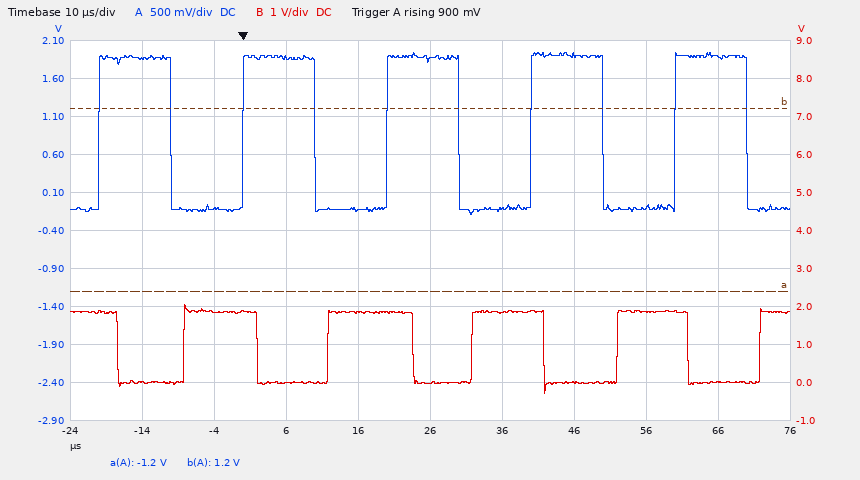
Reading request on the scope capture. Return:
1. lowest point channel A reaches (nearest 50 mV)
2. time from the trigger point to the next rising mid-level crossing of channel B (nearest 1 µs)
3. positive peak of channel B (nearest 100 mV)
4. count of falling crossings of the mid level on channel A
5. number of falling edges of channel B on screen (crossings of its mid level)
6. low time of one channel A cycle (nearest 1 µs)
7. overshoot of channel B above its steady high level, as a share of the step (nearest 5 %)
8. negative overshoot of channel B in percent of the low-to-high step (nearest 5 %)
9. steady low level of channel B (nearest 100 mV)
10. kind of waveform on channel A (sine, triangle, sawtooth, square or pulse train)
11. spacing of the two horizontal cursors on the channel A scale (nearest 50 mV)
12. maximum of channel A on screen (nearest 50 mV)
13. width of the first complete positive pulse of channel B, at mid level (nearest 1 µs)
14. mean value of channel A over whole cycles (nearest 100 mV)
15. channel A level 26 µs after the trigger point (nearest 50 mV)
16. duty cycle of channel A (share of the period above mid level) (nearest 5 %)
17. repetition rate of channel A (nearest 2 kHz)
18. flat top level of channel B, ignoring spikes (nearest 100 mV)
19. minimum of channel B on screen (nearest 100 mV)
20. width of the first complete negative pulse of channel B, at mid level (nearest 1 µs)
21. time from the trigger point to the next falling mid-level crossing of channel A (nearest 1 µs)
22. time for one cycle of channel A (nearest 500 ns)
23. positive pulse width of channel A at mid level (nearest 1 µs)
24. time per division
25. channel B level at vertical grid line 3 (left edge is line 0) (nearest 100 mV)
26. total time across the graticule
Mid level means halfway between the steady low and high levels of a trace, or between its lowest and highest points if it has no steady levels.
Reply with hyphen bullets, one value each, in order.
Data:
- -200 mV
- 12 µs
- 2.1 V
- 5
- 5
- 10 µs
- 10 %
- 15 %
- 0.0 V
- square
- 2.40 V
- 1.95 V
- 10 µs
- 900 mV
- 1.85 V
- 50 %
- 50 kHz
- 1.9 V
- -300 mV
- 9 µs
- 10 µs
- 20.0 µs
- 10 µs
- 10 µs
- 0.0 V
- 100 µs
